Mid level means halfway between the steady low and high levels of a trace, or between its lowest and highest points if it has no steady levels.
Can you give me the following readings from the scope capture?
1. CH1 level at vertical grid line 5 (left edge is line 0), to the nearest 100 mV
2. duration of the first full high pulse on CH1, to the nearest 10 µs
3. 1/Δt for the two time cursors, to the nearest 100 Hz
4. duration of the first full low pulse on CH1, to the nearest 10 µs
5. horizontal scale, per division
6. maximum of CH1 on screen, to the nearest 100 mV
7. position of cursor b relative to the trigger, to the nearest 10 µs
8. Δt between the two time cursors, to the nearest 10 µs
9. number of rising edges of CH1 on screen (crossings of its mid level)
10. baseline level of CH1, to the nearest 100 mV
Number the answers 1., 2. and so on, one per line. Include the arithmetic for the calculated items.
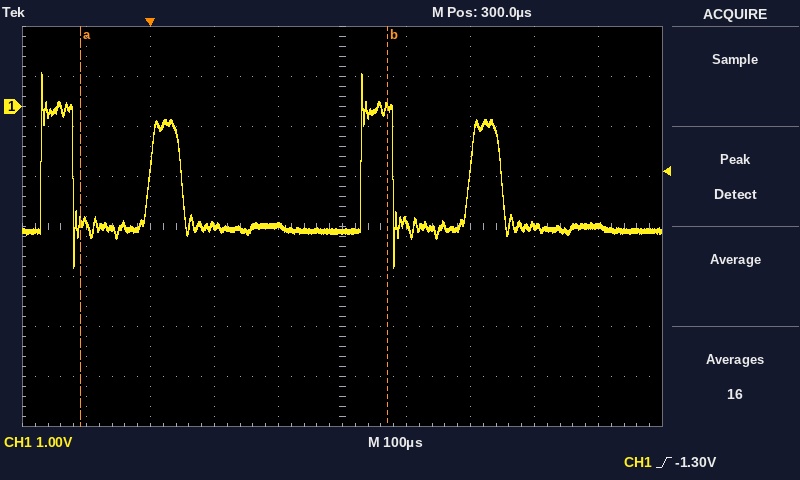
1. -2.5 V
2. 50 µs
3. 1 / 480 µs ≈ 2.1 kHz
4. 120 µs
5. 100 µs
6. 700 mV
7. +370 µs
8. 480 µs
9. 4
10. -2.5 V
